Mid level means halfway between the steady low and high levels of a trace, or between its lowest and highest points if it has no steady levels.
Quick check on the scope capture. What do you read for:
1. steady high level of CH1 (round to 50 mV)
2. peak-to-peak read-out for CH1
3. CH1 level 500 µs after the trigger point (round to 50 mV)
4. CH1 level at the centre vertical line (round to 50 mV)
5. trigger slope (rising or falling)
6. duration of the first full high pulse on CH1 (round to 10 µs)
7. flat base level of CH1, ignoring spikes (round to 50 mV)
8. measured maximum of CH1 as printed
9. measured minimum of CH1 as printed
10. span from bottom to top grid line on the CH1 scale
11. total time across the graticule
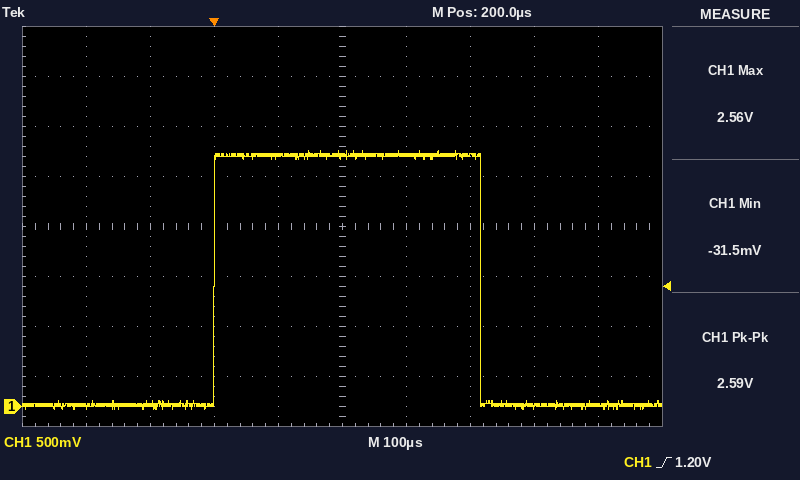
2.50 V
2.59 V
0 mV
2.50 V
rising
420 µs
0 mV
2.56 V
-31.5 mV
4 V
1 ms
